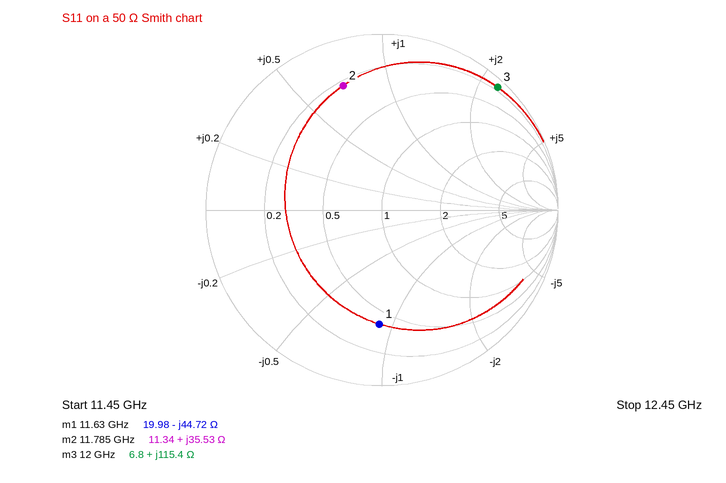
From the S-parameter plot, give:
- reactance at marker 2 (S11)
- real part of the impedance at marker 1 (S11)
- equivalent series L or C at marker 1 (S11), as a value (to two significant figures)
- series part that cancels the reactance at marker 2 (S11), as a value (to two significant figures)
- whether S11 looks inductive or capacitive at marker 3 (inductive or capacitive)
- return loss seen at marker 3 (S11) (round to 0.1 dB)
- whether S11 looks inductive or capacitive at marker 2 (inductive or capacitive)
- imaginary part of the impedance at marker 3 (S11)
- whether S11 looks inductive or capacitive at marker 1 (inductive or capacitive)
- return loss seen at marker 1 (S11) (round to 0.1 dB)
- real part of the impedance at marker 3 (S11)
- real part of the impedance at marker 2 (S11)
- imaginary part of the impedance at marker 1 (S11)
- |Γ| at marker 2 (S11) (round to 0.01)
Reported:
+35.53 Ω
19.98 Ω
310 fF
380 fF
inductive
0.4 dB
inductive
+115.4 Ω
capacitive
3.8 dB
6.8 Ω
11.34 Ω
-44.72 Ω
0.74
